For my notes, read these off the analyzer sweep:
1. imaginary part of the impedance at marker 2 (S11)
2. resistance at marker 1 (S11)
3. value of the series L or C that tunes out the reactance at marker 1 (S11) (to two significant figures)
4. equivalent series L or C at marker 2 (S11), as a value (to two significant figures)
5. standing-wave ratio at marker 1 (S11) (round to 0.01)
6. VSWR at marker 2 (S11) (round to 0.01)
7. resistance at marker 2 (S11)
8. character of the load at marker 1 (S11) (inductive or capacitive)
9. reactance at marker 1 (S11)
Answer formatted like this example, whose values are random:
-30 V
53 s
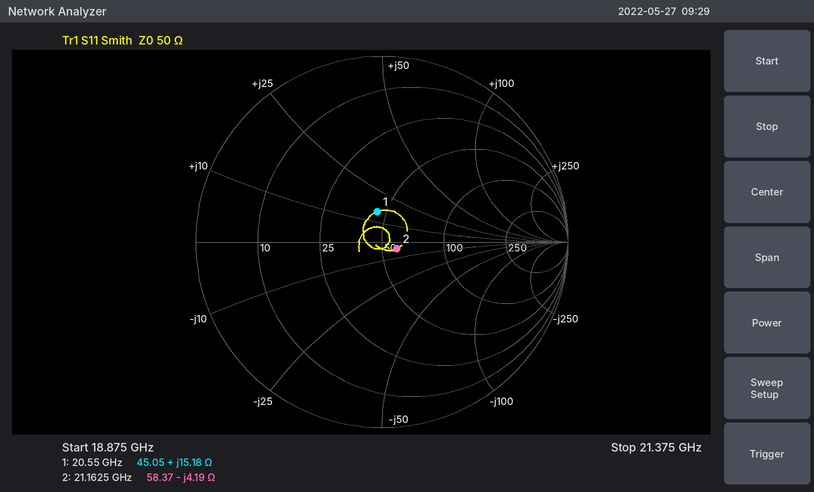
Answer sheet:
-4.19 Ω
45.05 Ω
510 fF
1.8 pF
1.40
1.19
58.37 Ω
inductive
+15.18 Ω
